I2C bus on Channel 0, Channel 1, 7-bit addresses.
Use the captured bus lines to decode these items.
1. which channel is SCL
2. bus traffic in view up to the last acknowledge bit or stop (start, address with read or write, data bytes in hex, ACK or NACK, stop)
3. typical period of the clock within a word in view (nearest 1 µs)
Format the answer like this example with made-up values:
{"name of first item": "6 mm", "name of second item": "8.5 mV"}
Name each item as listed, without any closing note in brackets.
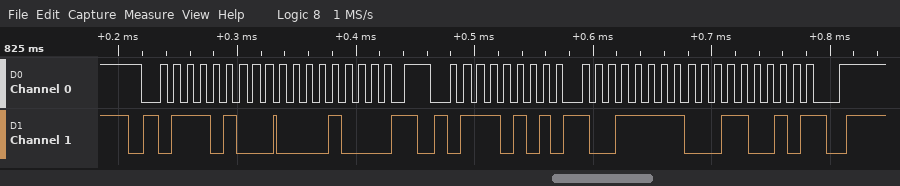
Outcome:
{"which channel is SCL": "Channel 0", "bus traffic in view up to the last acknowledge bit or stop": "start, address 3A write ACK, 08 ACK, repeated start, address 3A read ACK, 9F ACK, 32 NACK, stop", "typical period of the clock within a word in view": "11 µs"}
